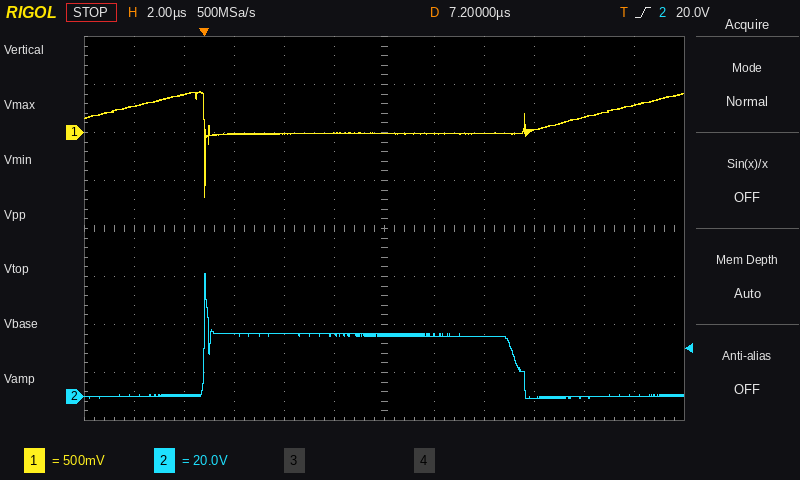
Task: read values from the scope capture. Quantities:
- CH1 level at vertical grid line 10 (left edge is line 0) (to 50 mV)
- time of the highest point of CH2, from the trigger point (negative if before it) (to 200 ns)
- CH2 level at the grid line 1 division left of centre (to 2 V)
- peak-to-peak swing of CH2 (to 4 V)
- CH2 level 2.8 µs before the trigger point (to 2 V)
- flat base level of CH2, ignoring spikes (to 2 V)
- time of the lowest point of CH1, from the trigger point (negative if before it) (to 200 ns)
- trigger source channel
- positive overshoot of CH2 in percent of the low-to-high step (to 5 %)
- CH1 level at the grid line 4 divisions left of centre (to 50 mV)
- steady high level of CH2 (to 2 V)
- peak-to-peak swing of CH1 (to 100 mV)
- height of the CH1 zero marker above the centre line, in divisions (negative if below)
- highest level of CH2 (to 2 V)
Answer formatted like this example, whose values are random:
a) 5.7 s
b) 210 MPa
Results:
a) 150 mV
b) 0.0 µs
c) 26 V
d) 52 V
e) 0 V
f) 0 V
g) 0.0 µs
h) CH2
i) 100 %
j) 400 mV
k) 26 V
l) 1.10 V
m) +2.0 div
n) 52 V
